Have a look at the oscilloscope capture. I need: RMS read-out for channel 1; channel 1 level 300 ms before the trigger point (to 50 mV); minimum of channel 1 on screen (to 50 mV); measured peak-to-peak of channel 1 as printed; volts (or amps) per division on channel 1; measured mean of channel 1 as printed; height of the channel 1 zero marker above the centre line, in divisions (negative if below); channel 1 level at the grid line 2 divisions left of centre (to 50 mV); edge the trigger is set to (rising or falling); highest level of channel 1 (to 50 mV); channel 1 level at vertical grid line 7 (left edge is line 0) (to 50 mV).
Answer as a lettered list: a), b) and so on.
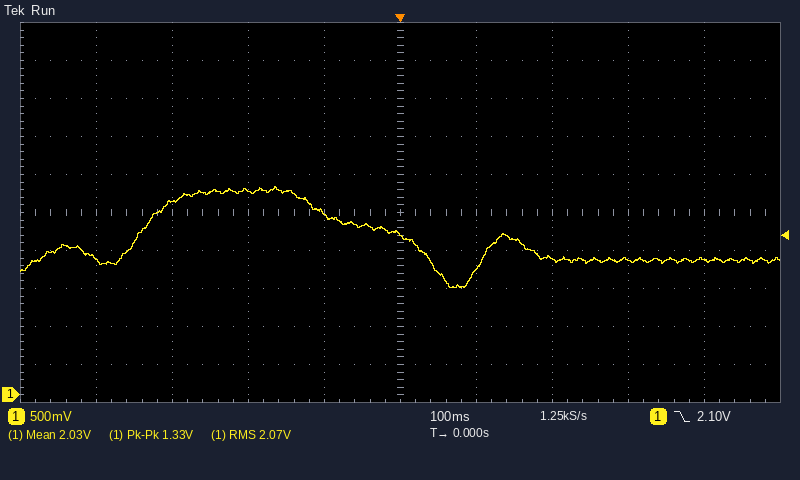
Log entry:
a) 2.07 V
b) 2.55 V
c) 1.40 V
d) 1.33 V
e) 500 mV
f) 2.03 V
g) -4.8 div
h) 2.70 V
i) falling
j) 2.75 V
k) 1.80 V
